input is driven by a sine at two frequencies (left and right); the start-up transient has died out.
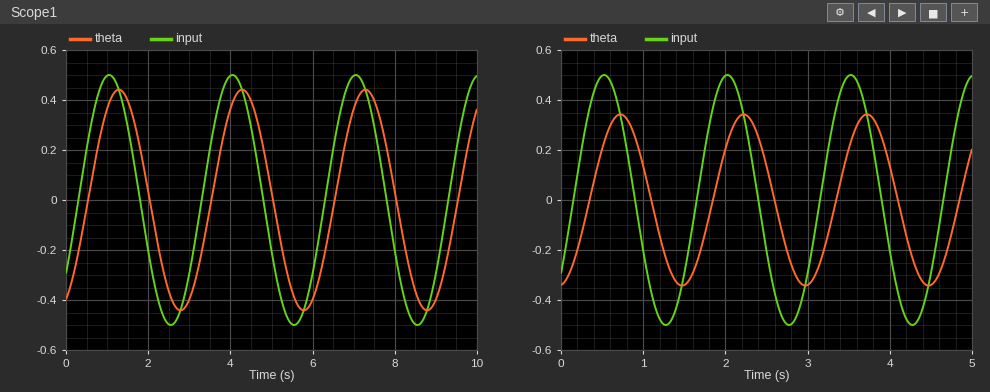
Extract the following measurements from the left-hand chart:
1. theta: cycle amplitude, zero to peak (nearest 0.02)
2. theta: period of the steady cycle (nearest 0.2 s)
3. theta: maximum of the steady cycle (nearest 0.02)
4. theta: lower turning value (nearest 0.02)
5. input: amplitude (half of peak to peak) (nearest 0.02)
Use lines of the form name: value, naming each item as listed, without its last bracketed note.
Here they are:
theta: cycle amplitude, zero to peak: 0.44
theta: period of the steady cycle: 3.0 s
theta: maximum of the steady cycle: 0.44
theta: lower turning value: -0.44
input: amplitude (half of peak to peak): 0.50
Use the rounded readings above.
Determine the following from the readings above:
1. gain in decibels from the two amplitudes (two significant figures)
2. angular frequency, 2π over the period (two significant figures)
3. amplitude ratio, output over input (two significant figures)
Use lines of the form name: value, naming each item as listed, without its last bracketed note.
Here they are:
gain in decibels from the two amplitudes: -1.1 dB
angular frequency, 2π over the period: 2.1 rad/s
amplitude ratio, output over input: 0.88
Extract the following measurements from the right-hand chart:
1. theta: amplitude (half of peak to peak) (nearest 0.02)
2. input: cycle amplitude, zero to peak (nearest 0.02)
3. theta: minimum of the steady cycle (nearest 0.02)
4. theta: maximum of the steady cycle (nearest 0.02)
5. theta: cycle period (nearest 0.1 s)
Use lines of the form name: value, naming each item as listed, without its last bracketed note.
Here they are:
theta: amplitude (half of peak to peak): 0.34
input: cycle amplitude, zero to peak: 0.50
theta: minimum of the steady cycle: -0.34
theta: maximum of the steady cycle: 0.34
theta: cycle period: 1.5 s
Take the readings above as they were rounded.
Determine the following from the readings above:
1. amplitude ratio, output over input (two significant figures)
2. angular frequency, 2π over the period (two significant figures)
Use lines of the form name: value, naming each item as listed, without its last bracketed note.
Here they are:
amplitude ratio, output over input: 0.68
angular frequency, 2π over the period: 4.2 rad/s
